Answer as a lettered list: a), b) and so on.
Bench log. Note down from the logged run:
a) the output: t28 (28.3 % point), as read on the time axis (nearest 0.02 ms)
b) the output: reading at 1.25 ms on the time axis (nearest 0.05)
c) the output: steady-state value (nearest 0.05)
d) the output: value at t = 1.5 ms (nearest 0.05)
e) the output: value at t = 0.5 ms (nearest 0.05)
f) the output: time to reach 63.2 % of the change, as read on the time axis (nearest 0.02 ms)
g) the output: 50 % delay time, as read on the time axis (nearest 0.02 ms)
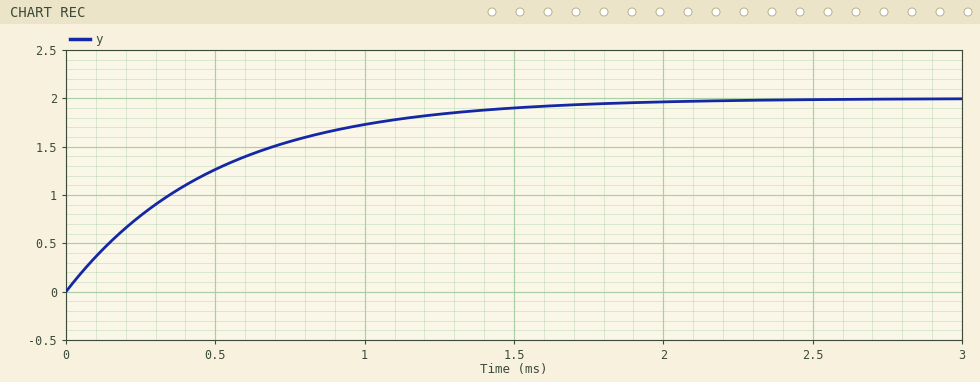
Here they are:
a) 0.16 ms
b) 1.85
c) 2.00
d) 1.90
e) 1.25
f) 0.50 ms
g) 0.34 ms
